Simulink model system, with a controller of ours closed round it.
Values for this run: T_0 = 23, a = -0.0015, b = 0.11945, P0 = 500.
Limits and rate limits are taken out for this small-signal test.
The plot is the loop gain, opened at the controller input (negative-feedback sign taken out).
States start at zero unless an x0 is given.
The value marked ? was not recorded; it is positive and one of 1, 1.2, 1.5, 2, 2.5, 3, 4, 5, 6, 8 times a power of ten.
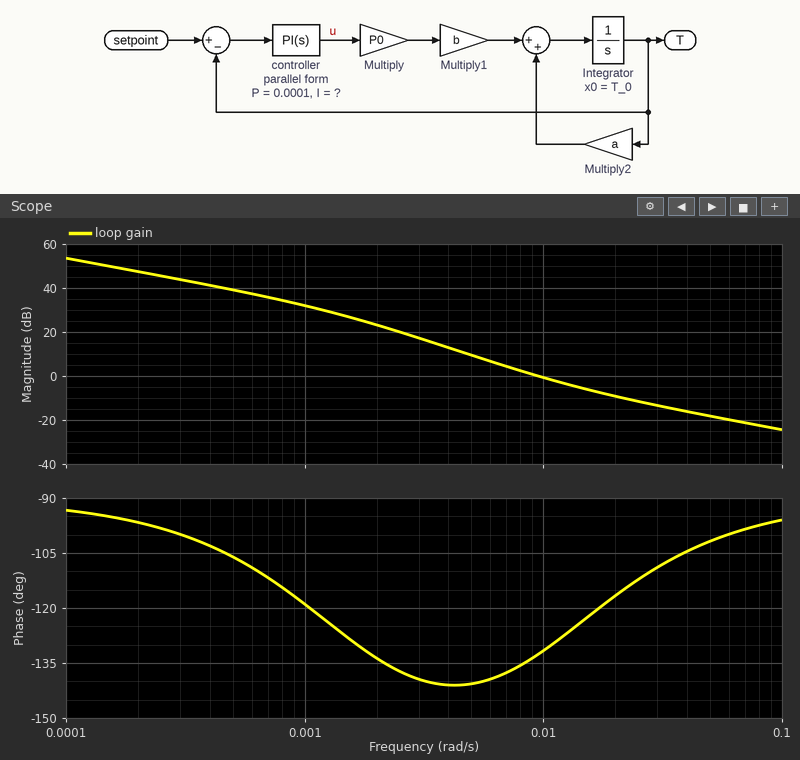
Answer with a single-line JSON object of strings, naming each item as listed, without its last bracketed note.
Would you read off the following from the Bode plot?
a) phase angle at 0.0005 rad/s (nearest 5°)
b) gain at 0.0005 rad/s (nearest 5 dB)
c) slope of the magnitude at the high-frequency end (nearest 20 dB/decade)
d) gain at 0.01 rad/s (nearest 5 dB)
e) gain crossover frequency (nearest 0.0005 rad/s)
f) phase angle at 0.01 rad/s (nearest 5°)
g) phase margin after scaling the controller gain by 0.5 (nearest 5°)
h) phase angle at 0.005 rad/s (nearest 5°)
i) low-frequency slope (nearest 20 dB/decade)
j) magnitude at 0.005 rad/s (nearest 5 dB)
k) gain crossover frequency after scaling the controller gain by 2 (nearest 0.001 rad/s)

{"phase angle at 0.0005 rad/s": "-105°", "gain at 0.0005 rad/s": "40 dB", "slope of the magnitude at the high-frequency end": "-20 dB/decade", "gain at 0.01 rad/s": "0 dB", "gain crossover frequency": "0.0095 rad/s", "phase angle at 0.01 rad/s": "-130°", "phase margin after scaling the controller gain by 0.5": "40°", "phase angle at 0.005 rad/s": "-140°", "low-frequency slope": "-20 dB/decade", "magnitude at 0.005 rad/s": "10 dB", "gain crossover frequency after scaling the controller gain by 2": "0.015 rad/s"}
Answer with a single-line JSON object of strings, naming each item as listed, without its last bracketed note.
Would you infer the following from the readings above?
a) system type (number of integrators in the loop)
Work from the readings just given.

{"system type": "1"}
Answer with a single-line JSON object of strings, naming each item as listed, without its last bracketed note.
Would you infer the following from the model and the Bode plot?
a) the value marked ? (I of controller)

{"the value marked ?": "1.2e-06"}
